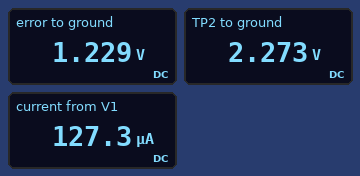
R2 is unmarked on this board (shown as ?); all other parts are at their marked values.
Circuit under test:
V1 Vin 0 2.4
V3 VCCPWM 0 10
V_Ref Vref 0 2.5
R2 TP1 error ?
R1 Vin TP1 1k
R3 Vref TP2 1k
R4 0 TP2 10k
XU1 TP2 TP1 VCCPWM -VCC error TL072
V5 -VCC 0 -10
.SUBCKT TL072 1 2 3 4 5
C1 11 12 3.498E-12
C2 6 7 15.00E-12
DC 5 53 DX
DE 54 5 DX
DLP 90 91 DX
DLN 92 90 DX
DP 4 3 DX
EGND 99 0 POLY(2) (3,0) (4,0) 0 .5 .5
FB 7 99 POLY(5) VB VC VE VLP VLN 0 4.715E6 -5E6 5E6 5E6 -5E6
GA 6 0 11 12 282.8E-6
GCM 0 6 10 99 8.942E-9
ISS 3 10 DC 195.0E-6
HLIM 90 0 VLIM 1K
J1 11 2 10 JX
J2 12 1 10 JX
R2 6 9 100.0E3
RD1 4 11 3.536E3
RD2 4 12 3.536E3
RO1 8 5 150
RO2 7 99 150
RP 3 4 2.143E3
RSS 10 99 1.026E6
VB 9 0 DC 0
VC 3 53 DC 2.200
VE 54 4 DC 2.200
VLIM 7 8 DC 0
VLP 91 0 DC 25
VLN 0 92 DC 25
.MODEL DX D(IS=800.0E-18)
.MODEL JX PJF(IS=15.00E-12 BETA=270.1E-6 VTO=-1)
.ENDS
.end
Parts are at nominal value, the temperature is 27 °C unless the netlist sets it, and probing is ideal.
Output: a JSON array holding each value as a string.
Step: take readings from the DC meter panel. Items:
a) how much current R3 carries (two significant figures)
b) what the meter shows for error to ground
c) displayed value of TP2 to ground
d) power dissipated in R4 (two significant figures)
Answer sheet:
["230 µA", "1.229 V", "2.273 V", "520 µW"]
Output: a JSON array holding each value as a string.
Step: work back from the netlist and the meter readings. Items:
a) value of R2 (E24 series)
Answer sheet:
["8.2 kΩ"]
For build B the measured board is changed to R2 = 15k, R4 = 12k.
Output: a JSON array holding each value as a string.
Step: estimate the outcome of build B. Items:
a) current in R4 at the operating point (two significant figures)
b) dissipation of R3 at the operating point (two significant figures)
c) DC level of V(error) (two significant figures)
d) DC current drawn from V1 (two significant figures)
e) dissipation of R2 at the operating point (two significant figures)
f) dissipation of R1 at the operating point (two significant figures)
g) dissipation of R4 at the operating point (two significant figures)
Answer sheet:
["190 µA", "37 µW", "920 mV", "92 µA", "130 µW", "8.5 µW", "440 µW"]
